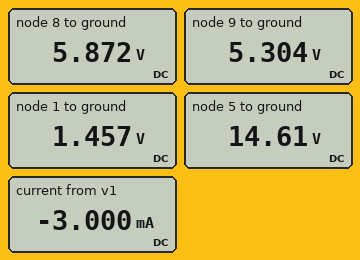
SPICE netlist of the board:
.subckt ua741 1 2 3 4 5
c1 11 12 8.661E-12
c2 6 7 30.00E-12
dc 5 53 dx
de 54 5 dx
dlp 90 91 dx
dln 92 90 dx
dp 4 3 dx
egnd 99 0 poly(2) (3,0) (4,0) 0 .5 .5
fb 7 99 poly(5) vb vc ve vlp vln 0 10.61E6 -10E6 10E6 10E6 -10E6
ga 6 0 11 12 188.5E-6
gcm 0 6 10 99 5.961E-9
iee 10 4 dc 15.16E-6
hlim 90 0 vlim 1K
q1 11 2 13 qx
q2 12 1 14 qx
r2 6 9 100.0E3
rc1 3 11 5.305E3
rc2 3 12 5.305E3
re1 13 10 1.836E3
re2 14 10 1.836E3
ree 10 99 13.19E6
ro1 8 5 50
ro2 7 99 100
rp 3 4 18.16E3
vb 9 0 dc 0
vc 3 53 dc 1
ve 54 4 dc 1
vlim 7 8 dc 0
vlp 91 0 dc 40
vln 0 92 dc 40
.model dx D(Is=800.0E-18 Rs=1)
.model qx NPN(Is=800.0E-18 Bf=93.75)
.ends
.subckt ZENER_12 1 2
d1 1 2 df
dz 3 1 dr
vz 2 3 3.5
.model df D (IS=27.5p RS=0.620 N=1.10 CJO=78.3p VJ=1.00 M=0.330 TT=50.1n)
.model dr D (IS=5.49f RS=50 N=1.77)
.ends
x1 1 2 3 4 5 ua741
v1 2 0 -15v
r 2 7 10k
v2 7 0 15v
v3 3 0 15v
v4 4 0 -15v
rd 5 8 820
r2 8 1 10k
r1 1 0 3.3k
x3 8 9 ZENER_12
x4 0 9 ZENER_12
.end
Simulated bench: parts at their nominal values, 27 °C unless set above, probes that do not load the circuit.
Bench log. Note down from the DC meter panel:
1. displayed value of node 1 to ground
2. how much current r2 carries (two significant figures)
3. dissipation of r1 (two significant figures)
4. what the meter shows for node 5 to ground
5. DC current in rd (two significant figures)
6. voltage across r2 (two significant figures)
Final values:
1.457 V
440 µA
640 µW
14.61 V
11 mA
4.4 V
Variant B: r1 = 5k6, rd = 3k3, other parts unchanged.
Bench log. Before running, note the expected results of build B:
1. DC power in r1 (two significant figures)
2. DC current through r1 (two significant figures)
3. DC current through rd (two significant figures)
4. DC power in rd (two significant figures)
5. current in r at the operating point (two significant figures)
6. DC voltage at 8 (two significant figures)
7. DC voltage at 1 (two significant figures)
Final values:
660 µW
340 µA
2.8 mA
26 mW
3.0 mA
5.4 V
1.9 V
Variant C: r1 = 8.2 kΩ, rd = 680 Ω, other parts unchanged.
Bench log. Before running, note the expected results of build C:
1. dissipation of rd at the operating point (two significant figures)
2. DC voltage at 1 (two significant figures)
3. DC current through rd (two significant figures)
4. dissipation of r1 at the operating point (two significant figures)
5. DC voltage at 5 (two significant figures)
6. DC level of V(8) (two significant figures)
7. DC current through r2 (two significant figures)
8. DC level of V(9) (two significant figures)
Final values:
110 mW
2.7 V
13 mA
890 µW
15 V
6.0 V
330 µA
5.4 V
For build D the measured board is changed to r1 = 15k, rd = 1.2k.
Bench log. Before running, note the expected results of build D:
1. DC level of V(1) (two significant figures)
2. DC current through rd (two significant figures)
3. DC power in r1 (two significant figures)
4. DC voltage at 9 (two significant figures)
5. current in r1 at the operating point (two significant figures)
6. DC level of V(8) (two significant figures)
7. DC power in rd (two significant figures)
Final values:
3.4 V
7.4 mA
780 µW
5.1 V
230 µA
5.7 V
66 mW
